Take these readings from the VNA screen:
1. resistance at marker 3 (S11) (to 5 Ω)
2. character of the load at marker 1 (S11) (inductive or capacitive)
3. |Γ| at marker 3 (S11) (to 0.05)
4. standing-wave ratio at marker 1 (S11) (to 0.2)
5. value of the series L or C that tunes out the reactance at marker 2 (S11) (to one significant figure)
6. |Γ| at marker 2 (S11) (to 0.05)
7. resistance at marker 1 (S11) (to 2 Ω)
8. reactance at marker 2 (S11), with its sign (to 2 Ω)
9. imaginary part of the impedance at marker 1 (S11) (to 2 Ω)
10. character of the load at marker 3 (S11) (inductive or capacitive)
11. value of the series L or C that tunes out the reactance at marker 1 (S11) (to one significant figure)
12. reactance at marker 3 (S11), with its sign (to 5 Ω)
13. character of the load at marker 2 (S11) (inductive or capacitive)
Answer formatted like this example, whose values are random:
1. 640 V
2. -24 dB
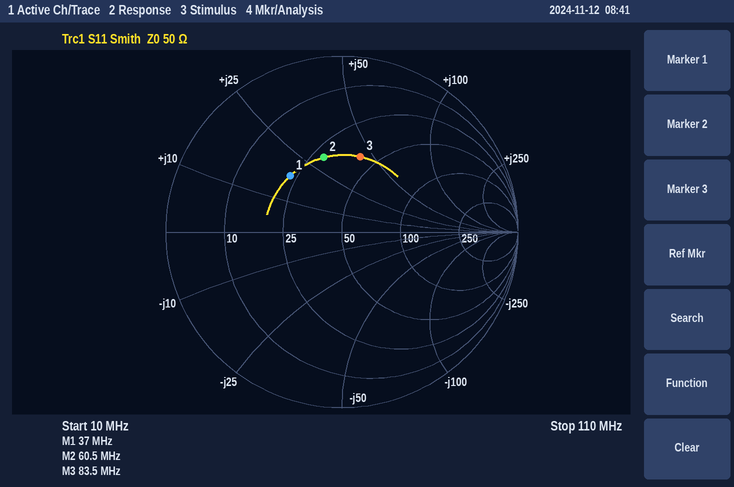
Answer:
1. 40 Ω
2. inductive
3. 0.45
4. 2.6
5. 90 pF
6. 0.45
7. 22 Ω
8. +30 Ω
9. +18 Ω
10. inductive
11. 200 pF
12. +45 Ω
13. inductive
